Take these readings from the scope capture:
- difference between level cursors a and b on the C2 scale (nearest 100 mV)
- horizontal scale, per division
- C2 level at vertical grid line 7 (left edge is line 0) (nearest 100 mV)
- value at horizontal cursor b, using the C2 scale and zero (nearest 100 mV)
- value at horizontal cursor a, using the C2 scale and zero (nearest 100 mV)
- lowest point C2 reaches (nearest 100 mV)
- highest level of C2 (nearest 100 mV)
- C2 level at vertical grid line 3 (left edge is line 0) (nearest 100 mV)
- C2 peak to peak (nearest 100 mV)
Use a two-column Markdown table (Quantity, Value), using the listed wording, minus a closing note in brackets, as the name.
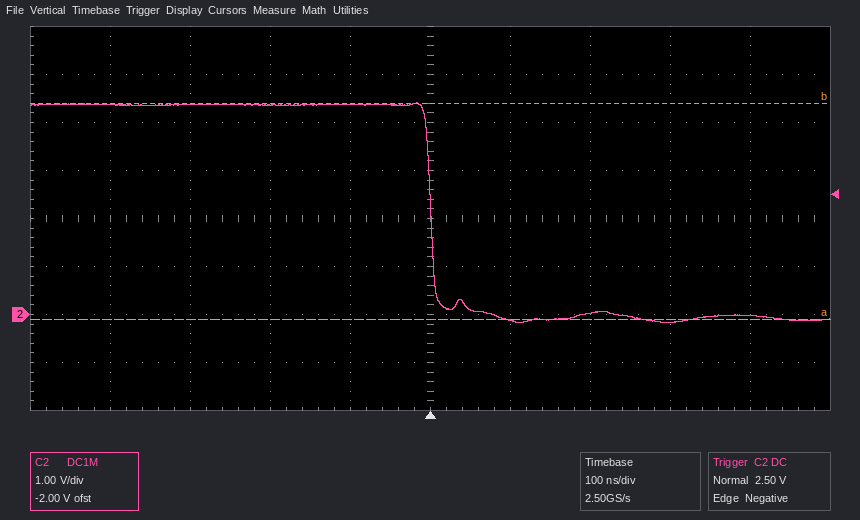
| Quantity | Value |
|---|---|
| difference between level cursors a and b on the C2 scale | 4.5 V |
| horizontal scale, per division | 100 ns |
| C2 level at vertical grid line 7 (left edge is line 0) | 0.0 V |
| value at horizontal cursor b, using the C2 scale and zero | 4.4 V |
| value at horizontal cursor a, using the C2 scale and zero | -100 mV |
| lowest point C2 reaches | -200 mV |
| highest level of C2 | 4.4 V |
| C2 level at vertical grid line 3 (left edge is line 0) | 4.4 V |
| C2 peak to peak | 4.6 V |
